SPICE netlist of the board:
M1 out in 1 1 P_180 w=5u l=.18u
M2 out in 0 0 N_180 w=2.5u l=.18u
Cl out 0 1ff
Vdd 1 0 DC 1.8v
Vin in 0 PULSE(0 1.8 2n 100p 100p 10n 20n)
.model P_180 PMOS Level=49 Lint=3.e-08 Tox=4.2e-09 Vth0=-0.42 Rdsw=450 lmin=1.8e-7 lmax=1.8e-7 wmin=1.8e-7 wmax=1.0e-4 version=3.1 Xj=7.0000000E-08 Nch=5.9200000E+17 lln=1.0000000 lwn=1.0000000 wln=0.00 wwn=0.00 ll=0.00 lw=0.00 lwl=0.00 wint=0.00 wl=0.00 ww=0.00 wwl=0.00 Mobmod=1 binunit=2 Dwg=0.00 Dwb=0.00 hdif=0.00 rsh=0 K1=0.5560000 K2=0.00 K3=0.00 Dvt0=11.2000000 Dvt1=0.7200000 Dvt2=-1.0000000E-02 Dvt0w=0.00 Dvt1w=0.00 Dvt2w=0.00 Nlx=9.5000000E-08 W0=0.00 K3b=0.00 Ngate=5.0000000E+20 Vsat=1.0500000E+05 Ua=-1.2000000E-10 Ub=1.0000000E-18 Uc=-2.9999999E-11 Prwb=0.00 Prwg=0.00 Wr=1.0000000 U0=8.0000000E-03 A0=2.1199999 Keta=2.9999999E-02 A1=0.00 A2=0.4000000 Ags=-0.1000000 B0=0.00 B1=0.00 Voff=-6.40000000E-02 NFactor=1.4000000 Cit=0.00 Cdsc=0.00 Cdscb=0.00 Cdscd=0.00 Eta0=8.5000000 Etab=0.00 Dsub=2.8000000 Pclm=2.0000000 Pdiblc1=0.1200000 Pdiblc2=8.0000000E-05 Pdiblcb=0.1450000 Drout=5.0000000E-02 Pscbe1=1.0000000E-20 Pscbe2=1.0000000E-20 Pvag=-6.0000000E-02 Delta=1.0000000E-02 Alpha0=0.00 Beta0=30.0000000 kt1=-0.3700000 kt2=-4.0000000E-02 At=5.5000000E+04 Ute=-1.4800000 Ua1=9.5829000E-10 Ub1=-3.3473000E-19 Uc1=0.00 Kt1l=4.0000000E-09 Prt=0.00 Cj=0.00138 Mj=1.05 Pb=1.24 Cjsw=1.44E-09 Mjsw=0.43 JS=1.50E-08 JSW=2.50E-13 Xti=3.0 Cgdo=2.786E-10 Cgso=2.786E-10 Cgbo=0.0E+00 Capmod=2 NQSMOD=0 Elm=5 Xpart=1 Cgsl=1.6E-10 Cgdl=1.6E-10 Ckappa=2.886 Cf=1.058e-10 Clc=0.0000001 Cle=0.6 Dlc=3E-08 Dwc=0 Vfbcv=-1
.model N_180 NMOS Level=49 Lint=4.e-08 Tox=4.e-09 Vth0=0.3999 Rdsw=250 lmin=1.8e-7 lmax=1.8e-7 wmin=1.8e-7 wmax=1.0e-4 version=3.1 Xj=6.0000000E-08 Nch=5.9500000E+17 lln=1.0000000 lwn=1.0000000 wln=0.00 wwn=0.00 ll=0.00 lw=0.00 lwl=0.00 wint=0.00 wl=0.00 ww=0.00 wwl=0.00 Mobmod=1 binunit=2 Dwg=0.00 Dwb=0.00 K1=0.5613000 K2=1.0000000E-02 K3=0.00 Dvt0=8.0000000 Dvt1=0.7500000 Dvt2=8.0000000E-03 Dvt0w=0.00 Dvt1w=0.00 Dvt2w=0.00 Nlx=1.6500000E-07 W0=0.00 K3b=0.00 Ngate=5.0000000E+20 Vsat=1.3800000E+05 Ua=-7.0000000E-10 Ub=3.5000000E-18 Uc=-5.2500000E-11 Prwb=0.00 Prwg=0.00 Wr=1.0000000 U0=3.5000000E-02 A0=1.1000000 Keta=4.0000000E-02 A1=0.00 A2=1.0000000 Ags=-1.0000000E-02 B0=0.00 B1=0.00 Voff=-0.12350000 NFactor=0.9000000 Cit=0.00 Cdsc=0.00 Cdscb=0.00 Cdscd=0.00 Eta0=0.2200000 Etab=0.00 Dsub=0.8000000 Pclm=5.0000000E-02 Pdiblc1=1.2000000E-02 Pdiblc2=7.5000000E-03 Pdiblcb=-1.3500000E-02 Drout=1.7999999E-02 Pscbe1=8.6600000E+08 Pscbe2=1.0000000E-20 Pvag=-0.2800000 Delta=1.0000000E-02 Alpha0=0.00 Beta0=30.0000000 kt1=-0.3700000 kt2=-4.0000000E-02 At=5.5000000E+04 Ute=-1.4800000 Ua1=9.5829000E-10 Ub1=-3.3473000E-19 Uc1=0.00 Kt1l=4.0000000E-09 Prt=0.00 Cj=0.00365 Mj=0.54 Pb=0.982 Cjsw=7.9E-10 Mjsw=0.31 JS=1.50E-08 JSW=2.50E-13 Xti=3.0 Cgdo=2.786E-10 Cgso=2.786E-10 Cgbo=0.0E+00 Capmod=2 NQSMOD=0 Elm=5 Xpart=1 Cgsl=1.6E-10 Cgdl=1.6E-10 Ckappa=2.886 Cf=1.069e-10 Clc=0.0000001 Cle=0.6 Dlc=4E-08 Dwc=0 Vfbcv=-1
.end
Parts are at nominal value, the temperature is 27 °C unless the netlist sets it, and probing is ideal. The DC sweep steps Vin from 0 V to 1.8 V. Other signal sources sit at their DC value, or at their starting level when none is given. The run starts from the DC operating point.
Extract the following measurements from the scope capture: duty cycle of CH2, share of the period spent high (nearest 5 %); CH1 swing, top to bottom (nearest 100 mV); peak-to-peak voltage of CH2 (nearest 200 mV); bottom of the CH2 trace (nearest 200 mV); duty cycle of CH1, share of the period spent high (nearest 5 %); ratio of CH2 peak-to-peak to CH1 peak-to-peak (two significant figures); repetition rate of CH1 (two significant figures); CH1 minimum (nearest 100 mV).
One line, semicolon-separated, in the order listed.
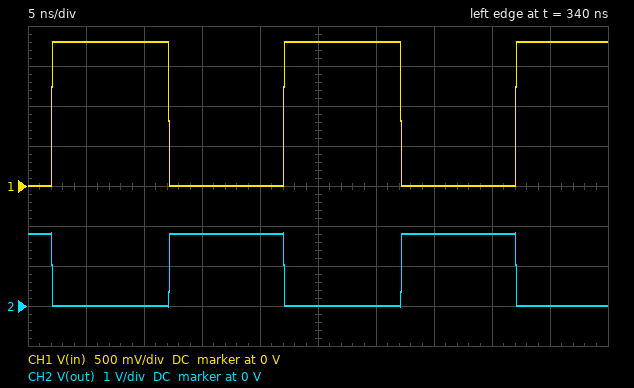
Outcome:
50 %; 1.8 V; 1.8 V; 0 V; 50 %; 1.0; 50 MHz; 0 V
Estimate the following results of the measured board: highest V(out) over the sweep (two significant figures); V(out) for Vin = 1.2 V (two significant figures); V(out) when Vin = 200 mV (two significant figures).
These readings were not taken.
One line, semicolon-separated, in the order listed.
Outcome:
1.8 V; 82 mV; 1.8 V
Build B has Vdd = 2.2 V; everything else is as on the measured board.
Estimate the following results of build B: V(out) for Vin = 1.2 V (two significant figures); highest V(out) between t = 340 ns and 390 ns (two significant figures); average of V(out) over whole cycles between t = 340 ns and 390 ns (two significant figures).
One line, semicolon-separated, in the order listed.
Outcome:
360 mV; 2.2 V; 1.1 V
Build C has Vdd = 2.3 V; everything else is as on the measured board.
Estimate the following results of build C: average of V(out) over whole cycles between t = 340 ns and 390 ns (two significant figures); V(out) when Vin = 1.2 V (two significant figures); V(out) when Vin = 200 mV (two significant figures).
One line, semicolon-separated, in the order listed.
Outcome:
1.2 V; 550 mV; 2.3 V
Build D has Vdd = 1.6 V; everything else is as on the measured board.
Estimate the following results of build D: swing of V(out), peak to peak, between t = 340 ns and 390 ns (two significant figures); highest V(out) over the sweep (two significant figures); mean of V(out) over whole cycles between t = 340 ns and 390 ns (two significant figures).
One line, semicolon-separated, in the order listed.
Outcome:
1.7 V; 1.6 V; 790 mV
